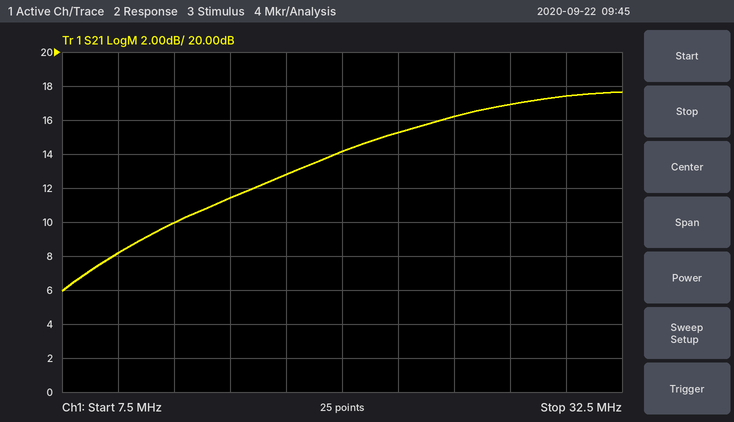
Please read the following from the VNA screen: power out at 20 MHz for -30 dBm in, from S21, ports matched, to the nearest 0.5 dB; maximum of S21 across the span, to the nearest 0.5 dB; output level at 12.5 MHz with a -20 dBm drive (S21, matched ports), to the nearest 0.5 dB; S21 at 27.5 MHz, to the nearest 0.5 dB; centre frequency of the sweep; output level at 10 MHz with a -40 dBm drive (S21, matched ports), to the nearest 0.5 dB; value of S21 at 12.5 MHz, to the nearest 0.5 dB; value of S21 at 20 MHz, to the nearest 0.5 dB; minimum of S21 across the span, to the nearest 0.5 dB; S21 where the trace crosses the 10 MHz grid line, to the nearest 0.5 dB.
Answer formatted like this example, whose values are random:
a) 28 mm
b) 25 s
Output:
a) -16.0 dBm
b) 17.5 dB
c) -10.0 dBm
d) 17.0 dB
e) 20 MHz
f) -32.0 dBm
g) 10.0 dB
h) 14.0 dB
i) 6.0 dB
j) 8.0 dB
